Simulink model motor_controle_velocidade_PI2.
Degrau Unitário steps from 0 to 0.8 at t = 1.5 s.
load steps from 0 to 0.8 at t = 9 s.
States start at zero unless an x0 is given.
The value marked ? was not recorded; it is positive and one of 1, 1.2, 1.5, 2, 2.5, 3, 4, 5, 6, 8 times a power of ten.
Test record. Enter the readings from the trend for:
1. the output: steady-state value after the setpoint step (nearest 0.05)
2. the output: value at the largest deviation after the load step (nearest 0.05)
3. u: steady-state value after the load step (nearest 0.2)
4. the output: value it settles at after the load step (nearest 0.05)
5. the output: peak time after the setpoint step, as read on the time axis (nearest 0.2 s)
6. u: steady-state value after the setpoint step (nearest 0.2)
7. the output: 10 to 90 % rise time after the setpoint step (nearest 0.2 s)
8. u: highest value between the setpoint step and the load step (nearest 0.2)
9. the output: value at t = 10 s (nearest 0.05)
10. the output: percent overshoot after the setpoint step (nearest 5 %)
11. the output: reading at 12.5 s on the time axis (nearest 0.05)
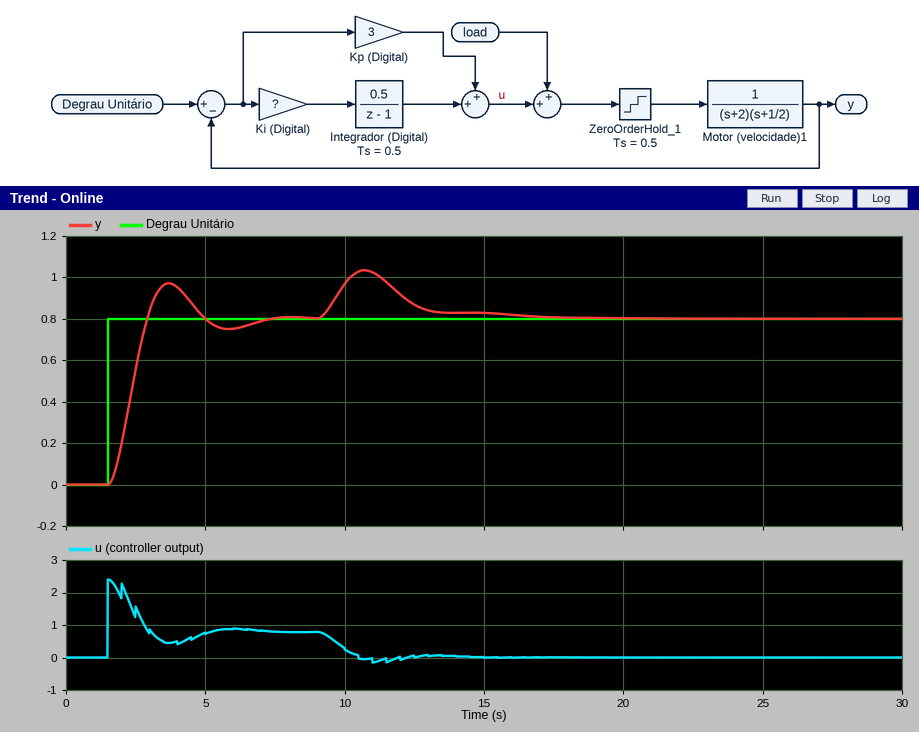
0.80
1.05
0.0
0.80
3.6 s
0.8
1.0 s
2.4
0.95
20 %
0.85
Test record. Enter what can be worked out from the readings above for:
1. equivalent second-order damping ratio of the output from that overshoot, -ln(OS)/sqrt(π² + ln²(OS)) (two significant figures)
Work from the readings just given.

0.46
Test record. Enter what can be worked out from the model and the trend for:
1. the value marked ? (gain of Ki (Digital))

1.2
